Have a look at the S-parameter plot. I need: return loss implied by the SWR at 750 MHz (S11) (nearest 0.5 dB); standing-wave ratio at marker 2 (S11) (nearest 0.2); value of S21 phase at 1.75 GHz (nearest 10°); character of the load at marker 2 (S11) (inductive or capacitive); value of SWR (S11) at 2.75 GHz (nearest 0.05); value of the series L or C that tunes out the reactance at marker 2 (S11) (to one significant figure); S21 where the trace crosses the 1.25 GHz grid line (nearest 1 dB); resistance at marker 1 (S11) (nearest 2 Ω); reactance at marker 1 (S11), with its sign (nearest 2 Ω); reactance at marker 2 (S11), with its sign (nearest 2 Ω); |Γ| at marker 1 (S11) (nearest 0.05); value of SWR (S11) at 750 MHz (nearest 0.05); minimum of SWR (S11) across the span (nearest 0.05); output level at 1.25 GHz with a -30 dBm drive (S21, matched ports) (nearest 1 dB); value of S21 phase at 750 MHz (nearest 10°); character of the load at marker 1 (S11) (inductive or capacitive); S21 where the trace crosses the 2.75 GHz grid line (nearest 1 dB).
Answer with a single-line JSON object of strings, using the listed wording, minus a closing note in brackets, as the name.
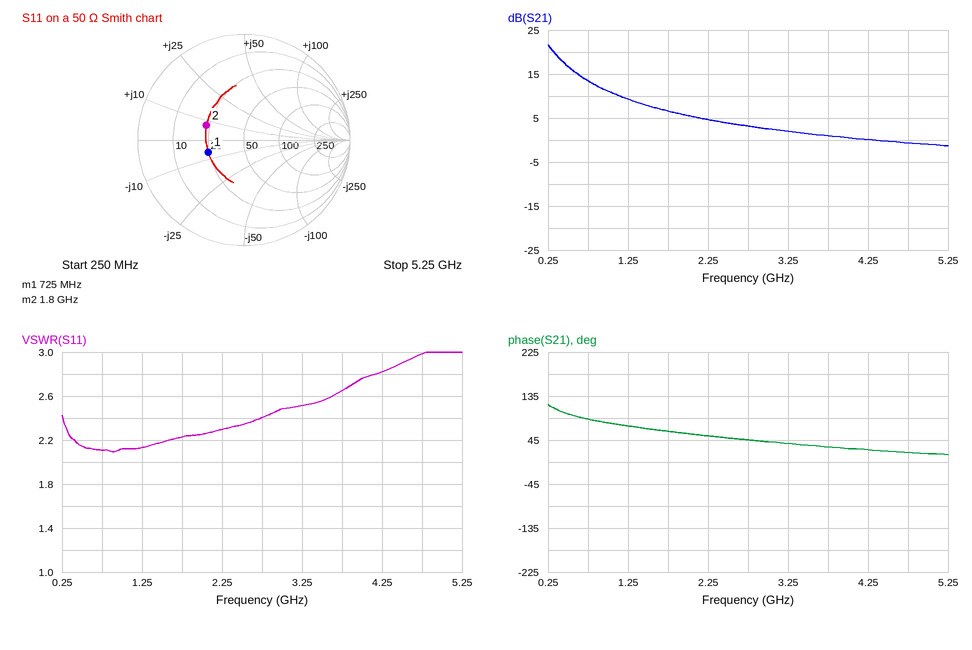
{"return loss implied by the SWR at 750 MHz (S11)": "9.0 dB", "standing-wave ratio at marker 2 (S11)": "2.2", "value of S21 phase at 1.75 GHz": "60°", "character of the load at marker 2 (S11)": "inductive", "value of SWR (S11) at 2.75 GHz": "2.40", "value of the series L or C that tunes out the reactance at marker 2 (S11)": "10 pF", "S21 where the trace crosses the 1.25 GHz grid line": "9 dB", "resistance at marker 1 (S11)": "24 Ω", "reactance at marker 1 (S11), with its sign": "-6 Ω", "reactance at marker 2 (S11), with its sign": "+8 Ω", "|Γ| at marker 1 (S11)": "0.35", "value of SWR (S11) at 750 MHz": "2.10", "minimum of SWR (S11) across the span": "2.10", "output level at 1.25 GHz with a -30 dBm drive (S21, matched ports)": "-21 dBm", "value of S21 phase at 750 MHz": "90°", "character of the load at marker 1 (S11)": "capacitive", "S21 where the trace crosses the 2.75 GHz grid line": "3 dB"}
